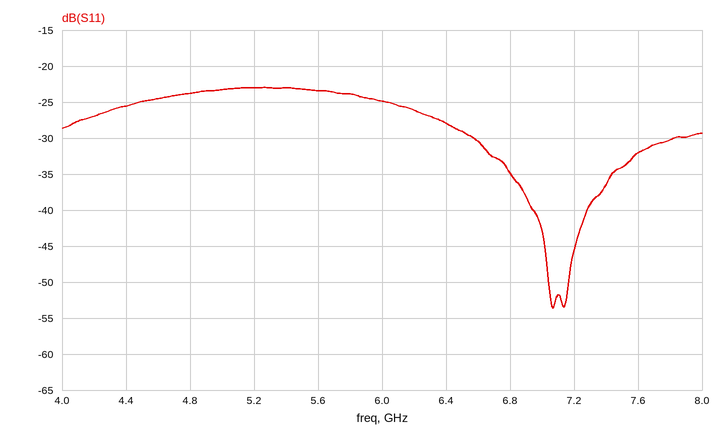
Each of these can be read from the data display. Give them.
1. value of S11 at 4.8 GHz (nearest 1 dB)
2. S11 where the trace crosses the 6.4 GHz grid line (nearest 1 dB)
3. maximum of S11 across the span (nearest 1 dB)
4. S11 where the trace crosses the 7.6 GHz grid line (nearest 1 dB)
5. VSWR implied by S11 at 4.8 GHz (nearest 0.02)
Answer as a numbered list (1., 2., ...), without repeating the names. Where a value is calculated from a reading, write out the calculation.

1. -24 dB
2. -28 dB
3. -23 dB
4. -32 dB
5. |Γ| = 10^(-24/20) = 0.0631; VSWR = (1 + 0.0631)/(1 − 0.0631) ≈ 1.13, so 1.14 to the nearest 0.02
